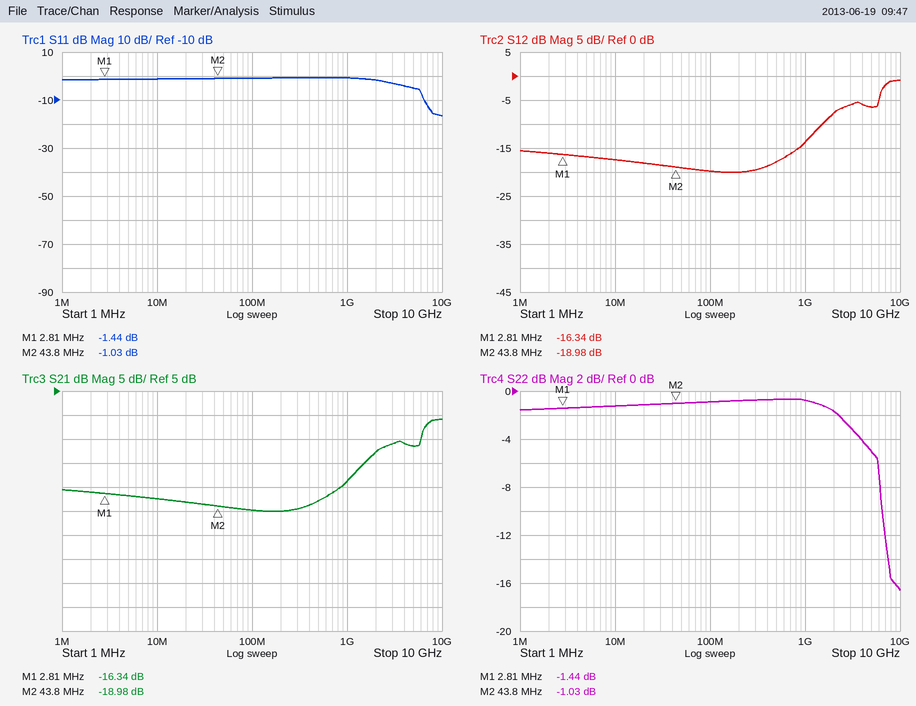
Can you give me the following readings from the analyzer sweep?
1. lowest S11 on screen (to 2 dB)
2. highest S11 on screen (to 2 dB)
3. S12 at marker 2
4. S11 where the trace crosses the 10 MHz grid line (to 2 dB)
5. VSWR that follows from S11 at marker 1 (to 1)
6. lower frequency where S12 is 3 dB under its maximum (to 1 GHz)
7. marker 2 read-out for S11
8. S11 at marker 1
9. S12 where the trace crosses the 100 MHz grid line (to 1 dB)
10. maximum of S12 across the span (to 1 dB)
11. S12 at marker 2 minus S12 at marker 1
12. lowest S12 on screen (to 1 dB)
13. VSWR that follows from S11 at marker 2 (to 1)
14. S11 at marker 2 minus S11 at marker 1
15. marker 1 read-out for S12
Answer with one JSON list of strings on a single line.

["-16 dB", "0 dB", "-18.98 dB", "-2 dB", "12", "6 GHz", "-1.03 dB", "-1.44 dB", "-20 dB", "-1 dB", "-2.64 dB", "-20 dB", "17", "0.41 dB", "-16.34 dB"]
